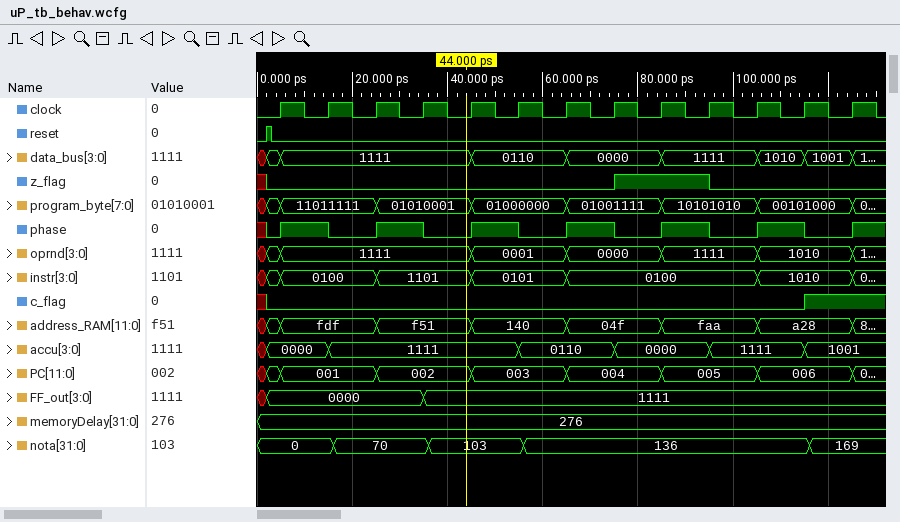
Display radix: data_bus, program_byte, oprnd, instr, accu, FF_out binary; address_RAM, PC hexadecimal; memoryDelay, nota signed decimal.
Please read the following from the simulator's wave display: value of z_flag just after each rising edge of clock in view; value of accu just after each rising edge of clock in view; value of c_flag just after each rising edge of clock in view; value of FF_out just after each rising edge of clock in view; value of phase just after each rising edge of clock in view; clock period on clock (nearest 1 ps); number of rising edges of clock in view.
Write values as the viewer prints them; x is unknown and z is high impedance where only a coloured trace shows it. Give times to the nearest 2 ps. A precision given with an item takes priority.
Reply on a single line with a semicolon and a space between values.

0 0 0 0 0 0 0 1 1 0 0 0 0; 0000, 1111, 1111, 1111, 1111, 0110, 0110, 0000, 0000, 1111, 1111, 1001, 1001; 0 0 0 0 0 0 0 0 0 0 0 1 1; 0000, 0000, 0000, 1111, 1111, 1111, 1111, 1111, 1111, 1111, 1111, 1111, 1111; 1 0 1 0 1 0 1 0 1 0 1 0 1; 10 ps; 13
